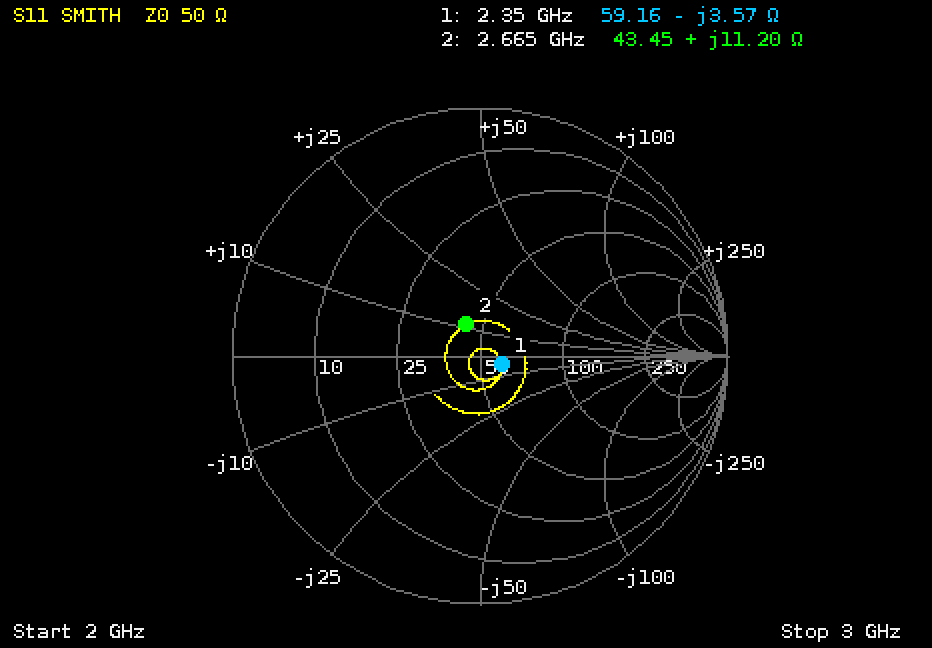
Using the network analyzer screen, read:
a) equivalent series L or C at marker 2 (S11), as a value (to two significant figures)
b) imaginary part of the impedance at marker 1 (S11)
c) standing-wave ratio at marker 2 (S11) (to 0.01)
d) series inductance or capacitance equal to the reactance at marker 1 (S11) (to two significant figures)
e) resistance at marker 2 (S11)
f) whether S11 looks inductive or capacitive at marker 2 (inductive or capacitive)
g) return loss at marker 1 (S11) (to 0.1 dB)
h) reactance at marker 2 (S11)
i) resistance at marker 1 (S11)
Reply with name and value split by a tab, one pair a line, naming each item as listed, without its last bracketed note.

equivalent series L or C at marker 2 (S11), as a value	670 pH
imaginary part of the impedance at marker 1	-3.57 Ω
standing-wave ratio at marker 2 (S11)	1.32
series inductance or capacitance equal to the reactance at marker 1 (S11)	19 pF
resistance at marker 2	43.45 Ω
whether S11 looks inductive or capacitive at marker 2	inductive
return loss at marker 1 (S11)	20.9 dB
reactance at marker 2	+11.20 Ω
resistance at marker 1	59.16 Ω
